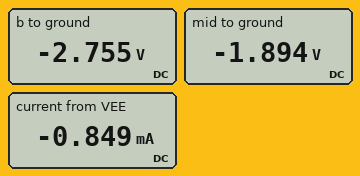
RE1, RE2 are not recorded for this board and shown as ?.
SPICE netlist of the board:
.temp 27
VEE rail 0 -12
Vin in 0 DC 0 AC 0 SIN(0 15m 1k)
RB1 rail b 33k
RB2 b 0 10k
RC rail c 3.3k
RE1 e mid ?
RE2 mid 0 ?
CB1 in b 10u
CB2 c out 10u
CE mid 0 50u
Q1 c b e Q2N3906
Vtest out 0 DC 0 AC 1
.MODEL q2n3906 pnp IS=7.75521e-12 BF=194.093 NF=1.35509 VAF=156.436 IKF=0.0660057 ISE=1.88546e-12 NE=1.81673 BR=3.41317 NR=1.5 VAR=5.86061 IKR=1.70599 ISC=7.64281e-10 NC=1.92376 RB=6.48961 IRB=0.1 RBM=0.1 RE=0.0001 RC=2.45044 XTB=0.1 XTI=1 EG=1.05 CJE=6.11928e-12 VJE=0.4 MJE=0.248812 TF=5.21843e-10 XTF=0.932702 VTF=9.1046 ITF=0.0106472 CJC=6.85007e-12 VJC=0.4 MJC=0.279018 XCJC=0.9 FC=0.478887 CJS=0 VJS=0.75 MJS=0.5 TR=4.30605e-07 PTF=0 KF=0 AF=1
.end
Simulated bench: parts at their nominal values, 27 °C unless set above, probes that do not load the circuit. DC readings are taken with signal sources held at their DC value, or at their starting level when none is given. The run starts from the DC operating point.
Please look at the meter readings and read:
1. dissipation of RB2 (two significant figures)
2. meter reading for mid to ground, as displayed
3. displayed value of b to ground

760 µW
-1.894 V
-2.755 V
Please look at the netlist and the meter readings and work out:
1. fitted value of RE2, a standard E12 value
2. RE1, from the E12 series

3.3 kΩ
390 Ω
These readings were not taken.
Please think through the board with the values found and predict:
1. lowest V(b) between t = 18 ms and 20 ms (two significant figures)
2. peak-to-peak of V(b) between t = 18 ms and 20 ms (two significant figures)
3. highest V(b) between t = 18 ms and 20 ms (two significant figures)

-2.8 V
30 mV
-2.7 V
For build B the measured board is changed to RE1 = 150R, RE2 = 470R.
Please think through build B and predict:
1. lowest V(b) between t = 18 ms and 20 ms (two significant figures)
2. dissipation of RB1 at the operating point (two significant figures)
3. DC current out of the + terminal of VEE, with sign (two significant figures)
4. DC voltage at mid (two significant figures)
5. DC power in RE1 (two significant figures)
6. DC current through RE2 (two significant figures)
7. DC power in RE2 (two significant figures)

-2.6 V
2.7 mW
-3.3 mA
-1.4 V
1.4 mW
3.0 mA
4.3 mW
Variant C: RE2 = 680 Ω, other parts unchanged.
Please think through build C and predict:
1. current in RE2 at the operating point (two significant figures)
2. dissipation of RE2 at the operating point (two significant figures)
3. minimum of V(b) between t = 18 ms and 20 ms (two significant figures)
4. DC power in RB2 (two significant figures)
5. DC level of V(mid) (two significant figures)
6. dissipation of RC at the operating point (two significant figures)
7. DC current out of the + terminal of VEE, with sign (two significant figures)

1.9 mA
2.4 mW
-2.7 V
720 µW
-1.3 V
11 mW
-2.1 mA
